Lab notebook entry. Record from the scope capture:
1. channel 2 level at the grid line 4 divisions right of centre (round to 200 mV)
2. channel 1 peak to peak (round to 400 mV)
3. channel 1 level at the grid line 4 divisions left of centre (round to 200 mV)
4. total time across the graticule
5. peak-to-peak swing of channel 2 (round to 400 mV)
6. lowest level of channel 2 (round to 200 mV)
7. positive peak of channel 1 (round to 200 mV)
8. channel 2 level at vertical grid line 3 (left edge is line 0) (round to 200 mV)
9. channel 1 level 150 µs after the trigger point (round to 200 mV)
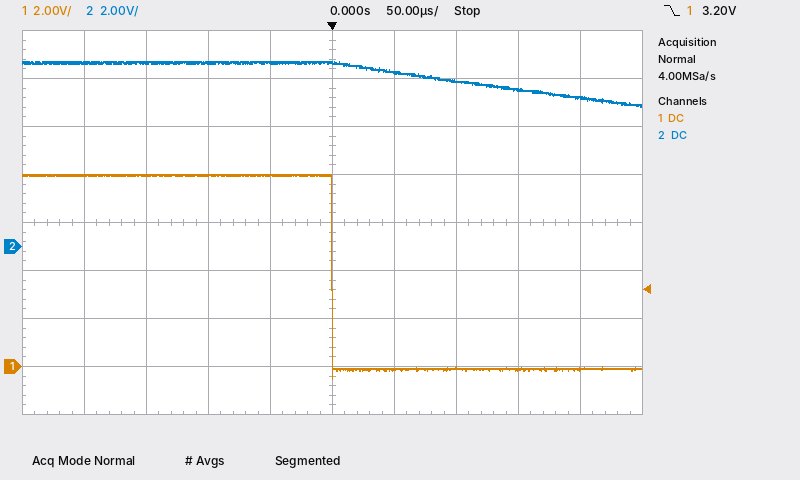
6.2 V
8.4 V
8.0 V
500 µs
2.0 V
5.8 V
8.0 V
7.6 V
-200 mV
